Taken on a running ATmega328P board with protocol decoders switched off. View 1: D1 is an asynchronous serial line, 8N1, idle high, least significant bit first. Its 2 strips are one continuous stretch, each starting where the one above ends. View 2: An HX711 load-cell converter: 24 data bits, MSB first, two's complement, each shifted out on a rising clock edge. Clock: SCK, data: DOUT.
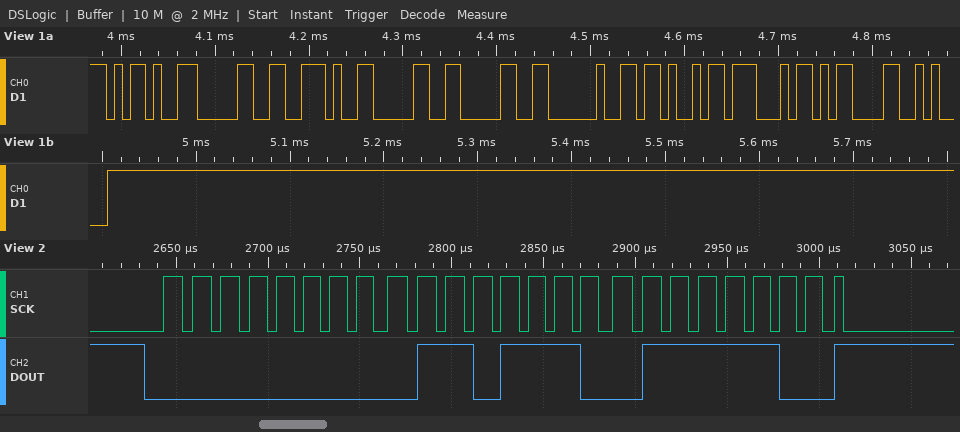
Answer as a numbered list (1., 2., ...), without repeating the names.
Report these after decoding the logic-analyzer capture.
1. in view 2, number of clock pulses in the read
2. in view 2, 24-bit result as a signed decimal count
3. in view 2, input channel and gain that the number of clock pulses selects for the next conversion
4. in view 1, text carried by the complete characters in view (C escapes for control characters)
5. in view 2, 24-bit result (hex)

1. 25
2. 28284
3. channel A, gain 128
4. "-0.00 KG\r\n"
5. 0x006E7C
